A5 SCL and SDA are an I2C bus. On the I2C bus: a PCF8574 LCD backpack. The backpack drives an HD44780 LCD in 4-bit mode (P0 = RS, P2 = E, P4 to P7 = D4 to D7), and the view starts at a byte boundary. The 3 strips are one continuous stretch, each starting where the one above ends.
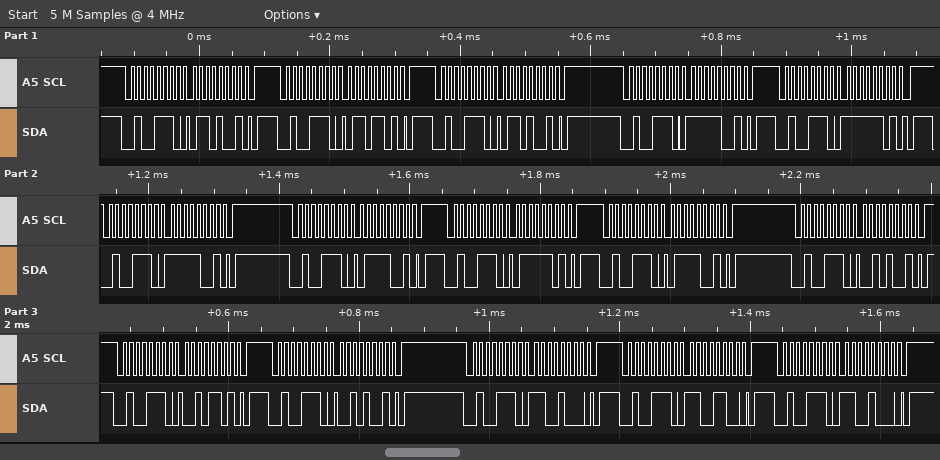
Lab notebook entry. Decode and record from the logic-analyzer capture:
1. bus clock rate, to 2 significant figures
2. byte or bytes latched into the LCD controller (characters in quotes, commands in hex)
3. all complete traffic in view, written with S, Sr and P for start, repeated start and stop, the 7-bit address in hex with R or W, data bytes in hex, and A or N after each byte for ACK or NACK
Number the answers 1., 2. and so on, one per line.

1. 100 kHz
2. 'o' 'r'
3. S 27W A 69 A P S 27W A 6D A P S 27W A 69 A P S 27W A F9 A P S 27W A FD A P S 27W A F9 A P S 27W A 79 A P S 27W A 7D A P S 27W A 79 A P S 27W A 29 A P S 27W A 2D A P S 27W A 29 A P S 27W A C8 A P S 27W A CC A P S 27W A C8 A P
